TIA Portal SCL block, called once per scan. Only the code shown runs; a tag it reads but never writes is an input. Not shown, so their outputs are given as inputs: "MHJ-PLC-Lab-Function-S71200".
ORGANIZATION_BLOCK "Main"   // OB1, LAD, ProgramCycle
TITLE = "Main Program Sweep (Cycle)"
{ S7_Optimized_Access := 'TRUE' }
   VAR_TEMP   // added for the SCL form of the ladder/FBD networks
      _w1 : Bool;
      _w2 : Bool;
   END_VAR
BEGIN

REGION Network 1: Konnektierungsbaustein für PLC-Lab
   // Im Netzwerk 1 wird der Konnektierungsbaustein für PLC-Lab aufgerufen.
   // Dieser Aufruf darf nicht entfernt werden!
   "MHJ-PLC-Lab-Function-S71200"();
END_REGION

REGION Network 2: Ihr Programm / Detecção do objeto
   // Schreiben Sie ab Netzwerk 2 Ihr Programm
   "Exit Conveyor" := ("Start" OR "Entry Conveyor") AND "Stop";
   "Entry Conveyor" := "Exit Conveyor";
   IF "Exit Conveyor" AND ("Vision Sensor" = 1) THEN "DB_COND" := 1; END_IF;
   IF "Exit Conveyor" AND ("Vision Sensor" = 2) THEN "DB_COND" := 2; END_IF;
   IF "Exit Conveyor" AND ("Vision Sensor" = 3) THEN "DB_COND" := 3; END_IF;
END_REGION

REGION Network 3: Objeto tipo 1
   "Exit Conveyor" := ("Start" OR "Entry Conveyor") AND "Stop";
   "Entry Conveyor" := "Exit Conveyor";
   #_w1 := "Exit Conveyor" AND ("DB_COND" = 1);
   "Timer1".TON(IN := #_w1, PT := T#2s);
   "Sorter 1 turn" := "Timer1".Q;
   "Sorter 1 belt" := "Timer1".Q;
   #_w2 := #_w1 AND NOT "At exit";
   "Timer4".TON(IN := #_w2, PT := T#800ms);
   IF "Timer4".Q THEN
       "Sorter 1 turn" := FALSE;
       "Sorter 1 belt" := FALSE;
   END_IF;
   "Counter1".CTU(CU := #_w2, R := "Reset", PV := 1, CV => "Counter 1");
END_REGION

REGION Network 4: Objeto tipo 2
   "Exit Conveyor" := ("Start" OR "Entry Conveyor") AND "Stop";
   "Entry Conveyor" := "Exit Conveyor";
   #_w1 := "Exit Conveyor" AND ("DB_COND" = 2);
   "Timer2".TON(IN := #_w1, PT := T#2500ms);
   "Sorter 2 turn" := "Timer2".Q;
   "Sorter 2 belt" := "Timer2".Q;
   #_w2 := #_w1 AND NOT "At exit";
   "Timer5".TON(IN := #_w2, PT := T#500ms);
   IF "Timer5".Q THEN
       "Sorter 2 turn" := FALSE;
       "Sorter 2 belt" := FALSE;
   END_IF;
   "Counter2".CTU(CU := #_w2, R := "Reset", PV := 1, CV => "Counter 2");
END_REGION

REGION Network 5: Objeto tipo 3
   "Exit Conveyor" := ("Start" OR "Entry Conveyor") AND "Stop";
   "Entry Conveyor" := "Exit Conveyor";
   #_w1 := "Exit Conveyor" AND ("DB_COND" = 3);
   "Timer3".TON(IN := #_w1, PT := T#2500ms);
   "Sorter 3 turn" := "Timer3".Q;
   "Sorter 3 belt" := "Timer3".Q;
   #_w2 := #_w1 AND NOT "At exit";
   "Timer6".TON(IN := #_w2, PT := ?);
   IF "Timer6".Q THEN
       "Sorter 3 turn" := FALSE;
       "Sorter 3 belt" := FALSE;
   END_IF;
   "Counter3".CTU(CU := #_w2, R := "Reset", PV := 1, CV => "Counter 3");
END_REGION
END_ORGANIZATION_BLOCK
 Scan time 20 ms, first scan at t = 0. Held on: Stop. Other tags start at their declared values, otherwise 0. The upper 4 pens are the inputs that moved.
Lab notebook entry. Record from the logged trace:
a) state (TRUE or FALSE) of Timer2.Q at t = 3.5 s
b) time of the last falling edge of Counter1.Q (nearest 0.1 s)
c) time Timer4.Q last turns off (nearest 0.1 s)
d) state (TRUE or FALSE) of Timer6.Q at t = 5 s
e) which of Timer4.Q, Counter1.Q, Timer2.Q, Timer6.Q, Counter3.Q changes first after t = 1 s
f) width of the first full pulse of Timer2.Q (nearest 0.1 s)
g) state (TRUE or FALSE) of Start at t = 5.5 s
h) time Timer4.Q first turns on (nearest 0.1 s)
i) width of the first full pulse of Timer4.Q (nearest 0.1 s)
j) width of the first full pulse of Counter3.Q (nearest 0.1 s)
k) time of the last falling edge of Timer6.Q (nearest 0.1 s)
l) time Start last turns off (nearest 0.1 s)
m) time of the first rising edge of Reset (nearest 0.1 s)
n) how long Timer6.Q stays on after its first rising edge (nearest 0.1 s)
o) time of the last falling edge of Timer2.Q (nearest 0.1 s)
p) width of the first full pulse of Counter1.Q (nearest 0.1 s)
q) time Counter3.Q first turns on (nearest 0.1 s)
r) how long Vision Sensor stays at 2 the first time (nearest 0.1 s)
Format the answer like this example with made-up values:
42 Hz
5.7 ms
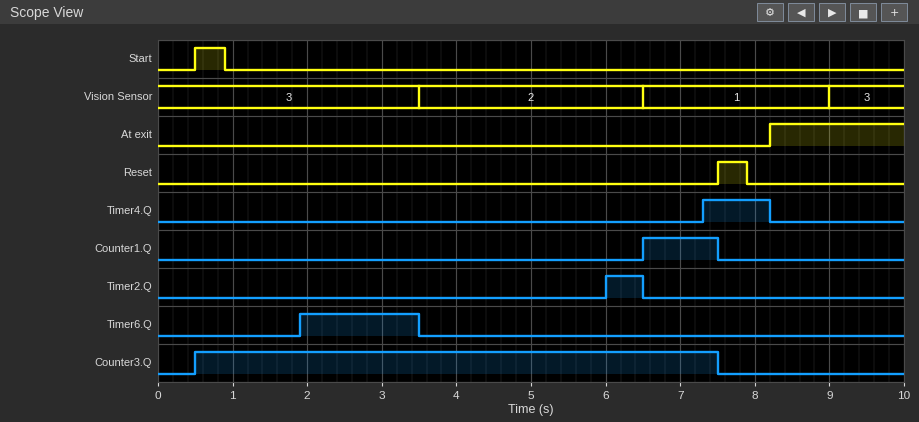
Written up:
FALSE
7.5 s
8.2 s
FALSE
Timer6.Q
0.5 s
FALSE
7.3 s
0.9 s
7.0 s
3.5 s
0.9 s
7.5 s
1.6 s
6.5 s
1.0 s
0.5 s
3.0 s
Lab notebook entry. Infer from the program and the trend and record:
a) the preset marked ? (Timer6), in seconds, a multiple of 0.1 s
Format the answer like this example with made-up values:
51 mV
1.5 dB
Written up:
1.4 s
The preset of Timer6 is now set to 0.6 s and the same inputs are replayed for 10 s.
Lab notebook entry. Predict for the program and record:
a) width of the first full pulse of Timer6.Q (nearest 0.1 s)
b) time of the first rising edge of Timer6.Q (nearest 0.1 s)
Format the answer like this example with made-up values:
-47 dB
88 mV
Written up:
2.4 s
1.1 s
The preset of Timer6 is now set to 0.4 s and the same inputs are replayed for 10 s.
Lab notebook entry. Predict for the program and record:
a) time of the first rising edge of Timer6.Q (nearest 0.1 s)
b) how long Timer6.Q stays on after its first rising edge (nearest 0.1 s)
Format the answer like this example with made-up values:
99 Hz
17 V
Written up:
0.9 s
2.6 s
